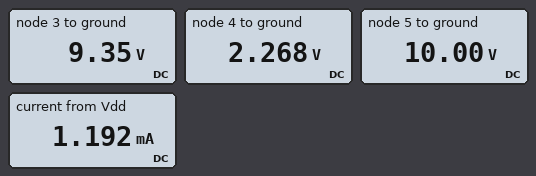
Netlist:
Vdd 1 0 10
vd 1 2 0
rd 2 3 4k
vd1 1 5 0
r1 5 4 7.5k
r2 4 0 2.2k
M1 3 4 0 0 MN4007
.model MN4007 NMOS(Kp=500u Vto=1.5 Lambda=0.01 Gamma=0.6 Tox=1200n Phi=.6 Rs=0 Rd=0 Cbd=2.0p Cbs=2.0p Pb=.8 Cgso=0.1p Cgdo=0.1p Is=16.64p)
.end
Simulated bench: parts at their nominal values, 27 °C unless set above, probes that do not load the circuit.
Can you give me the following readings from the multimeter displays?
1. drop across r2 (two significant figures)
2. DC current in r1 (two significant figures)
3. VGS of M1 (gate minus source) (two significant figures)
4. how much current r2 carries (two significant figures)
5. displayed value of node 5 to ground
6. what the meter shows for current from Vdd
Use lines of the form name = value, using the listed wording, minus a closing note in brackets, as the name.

drop across r2 = 2.3 V
DC current in r1 = 1.0 mA
VGS of M1 (gate minus source) = 2.3 V
how much current r2 carries = 1.0 mA
displayed value of node 5 to ground = 10.00 V
what the meter shows for current from Vdd = 1.192 mA
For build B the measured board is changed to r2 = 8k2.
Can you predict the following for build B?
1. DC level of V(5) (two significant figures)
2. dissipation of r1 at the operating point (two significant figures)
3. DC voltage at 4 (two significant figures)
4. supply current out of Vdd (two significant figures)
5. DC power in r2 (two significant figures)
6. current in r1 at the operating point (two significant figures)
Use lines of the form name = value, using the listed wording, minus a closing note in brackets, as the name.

DC level of V(5) = 10 V
dissipation of r1 at the operating point = 3.0 mW
DC voltage at 4 = 5.2 V
supply current out of Vdd = 2.8 mA
DC power in r2 = 3.3 mW
current in r1 at the operating point = 640 µA
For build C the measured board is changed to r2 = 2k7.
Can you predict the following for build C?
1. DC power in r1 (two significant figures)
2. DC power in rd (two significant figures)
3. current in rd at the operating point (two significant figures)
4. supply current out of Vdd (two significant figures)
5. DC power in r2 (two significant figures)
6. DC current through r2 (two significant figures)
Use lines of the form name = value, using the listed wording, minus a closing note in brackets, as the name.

DC power in r1 = 7.2 mW
DC power in rd = 510 µW
current in rd at the operating point = 360 µA
supply current out of Vdd = 1.3 mA
DC power in r2 = 2.6 mW
DC current through r2 = 980 µA
